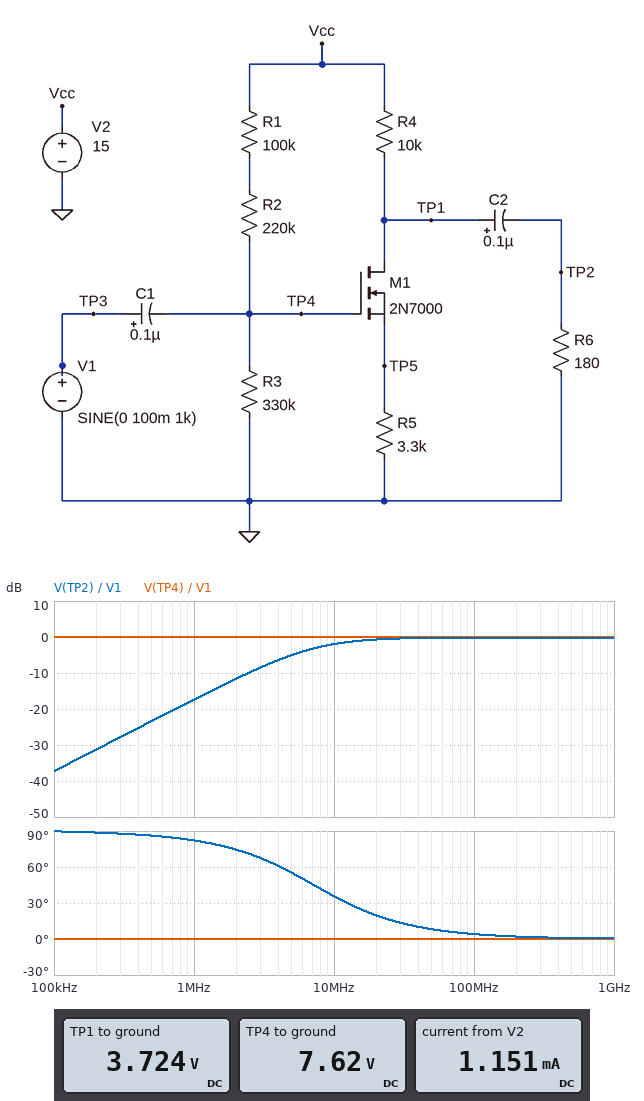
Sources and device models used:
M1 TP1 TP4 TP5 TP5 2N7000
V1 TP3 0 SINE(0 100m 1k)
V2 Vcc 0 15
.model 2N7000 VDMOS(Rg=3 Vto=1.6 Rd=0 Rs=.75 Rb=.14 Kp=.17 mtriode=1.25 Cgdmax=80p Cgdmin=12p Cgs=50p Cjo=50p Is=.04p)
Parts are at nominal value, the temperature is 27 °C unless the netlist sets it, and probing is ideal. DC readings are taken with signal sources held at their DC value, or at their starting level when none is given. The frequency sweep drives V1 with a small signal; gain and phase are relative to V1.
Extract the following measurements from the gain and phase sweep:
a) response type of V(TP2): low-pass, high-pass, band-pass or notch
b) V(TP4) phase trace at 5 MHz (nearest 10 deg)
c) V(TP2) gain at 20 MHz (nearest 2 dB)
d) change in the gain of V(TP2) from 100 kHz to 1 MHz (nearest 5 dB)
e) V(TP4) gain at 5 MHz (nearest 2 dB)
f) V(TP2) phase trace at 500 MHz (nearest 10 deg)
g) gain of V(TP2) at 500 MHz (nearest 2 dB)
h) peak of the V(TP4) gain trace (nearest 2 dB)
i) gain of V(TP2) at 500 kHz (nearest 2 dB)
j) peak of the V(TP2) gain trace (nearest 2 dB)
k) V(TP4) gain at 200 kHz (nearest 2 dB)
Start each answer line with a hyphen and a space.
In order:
- high-pass
- 0 deg
- 0 dB
- 20 dB
- 0 dB
- 0 deg
- 0 dB
- 0 dB
- -24 dB
- 0 dB
- 0 dB
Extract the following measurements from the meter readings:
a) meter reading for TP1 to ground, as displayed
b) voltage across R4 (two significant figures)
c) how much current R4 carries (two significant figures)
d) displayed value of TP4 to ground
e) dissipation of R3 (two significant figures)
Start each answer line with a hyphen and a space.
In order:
- 3.724 V
- 11 V
- 1.1 mA
- 7.62 V
- 180 µW
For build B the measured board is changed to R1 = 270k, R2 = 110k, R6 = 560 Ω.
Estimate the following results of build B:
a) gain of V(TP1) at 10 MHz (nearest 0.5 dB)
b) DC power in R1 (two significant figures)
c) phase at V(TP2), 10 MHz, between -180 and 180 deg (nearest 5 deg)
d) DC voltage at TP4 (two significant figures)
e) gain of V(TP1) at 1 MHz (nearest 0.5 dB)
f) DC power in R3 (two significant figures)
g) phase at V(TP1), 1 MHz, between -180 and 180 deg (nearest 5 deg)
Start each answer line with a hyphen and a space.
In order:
- -0.5 dB
- 120 µW
- 15 deg
- 7.0 V
- -9.0 dB
- 150 µW
- 70 deg
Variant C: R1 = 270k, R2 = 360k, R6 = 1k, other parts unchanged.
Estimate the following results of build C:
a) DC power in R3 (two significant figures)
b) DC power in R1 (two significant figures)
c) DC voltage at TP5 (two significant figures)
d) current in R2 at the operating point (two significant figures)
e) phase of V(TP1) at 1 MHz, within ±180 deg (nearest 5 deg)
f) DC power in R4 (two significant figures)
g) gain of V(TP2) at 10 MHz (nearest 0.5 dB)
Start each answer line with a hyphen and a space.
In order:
- 81 µW
- 66 µW
- 3.5 V
- 16 µA
- 100 deg
- 11 mW
- 0 dB
